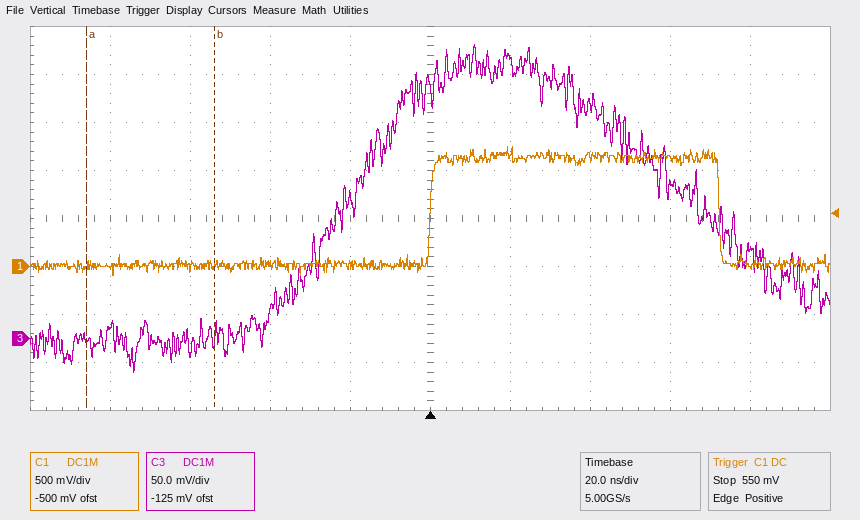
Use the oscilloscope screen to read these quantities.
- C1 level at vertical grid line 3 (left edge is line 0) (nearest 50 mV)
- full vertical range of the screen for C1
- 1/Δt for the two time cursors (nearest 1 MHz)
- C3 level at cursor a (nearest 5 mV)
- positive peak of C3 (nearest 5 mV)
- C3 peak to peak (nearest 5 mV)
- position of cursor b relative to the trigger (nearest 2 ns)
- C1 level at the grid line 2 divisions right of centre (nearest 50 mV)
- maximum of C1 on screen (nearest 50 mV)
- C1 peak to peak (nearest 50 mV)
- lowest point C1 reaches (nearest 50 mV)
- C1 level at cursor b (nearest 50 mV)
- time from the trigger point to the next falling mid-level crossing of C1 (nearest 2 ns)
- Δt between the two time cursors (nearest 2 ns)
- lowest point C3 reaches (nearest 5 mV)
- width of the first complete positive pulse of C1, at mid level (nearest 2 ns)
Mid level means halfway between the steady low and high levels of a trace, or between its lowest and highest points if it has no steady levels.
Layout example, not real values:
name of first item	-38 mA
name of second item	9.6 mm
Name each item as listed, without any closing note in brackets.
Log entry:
C1 level at vertical grid line 3 (left edge is line 0)	0 mV
full vertical range of the screen for C1	4 V
1/Δt for the two time cursors	31 MHz
C3 level at cursor a	0 mV
positive peak of C3	305 mV
C3 peak to peak	340 mV
position of cursor b relative to the trigger	-54 ns
C1 level at the grid line 2 divisions right of centre	1.15 V
maximum of C1 on screen	1.25 V
C1 peak to peak	1.35 V
lowest point C1 reaches	-100 mV
C1 level at cursor b	0 mV
time from the trigger point to the next falling mid-level crossing of C1	72 ns
Δt between the two time cursors	32 ns
lowest point C3 reaches	-35 mV
width of the first complete positive pulse of C1, at mid level	72 ns
